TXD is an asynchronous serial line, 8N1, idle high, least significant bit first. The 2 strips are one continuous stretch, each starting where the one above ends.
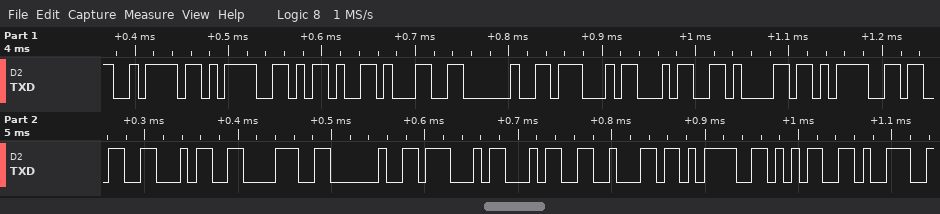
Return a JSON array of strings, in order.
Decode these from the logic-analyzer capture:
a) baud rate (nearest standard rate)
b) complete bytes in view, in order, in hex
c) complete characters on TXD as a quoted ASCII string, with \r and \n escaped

["115200 baud", "7A 3D 2D 31 20 47 34 61 3D 33 34 38 20 47 34 62 3D 35 39", "\"z=-1 G4a=348 G4b=59\""]
